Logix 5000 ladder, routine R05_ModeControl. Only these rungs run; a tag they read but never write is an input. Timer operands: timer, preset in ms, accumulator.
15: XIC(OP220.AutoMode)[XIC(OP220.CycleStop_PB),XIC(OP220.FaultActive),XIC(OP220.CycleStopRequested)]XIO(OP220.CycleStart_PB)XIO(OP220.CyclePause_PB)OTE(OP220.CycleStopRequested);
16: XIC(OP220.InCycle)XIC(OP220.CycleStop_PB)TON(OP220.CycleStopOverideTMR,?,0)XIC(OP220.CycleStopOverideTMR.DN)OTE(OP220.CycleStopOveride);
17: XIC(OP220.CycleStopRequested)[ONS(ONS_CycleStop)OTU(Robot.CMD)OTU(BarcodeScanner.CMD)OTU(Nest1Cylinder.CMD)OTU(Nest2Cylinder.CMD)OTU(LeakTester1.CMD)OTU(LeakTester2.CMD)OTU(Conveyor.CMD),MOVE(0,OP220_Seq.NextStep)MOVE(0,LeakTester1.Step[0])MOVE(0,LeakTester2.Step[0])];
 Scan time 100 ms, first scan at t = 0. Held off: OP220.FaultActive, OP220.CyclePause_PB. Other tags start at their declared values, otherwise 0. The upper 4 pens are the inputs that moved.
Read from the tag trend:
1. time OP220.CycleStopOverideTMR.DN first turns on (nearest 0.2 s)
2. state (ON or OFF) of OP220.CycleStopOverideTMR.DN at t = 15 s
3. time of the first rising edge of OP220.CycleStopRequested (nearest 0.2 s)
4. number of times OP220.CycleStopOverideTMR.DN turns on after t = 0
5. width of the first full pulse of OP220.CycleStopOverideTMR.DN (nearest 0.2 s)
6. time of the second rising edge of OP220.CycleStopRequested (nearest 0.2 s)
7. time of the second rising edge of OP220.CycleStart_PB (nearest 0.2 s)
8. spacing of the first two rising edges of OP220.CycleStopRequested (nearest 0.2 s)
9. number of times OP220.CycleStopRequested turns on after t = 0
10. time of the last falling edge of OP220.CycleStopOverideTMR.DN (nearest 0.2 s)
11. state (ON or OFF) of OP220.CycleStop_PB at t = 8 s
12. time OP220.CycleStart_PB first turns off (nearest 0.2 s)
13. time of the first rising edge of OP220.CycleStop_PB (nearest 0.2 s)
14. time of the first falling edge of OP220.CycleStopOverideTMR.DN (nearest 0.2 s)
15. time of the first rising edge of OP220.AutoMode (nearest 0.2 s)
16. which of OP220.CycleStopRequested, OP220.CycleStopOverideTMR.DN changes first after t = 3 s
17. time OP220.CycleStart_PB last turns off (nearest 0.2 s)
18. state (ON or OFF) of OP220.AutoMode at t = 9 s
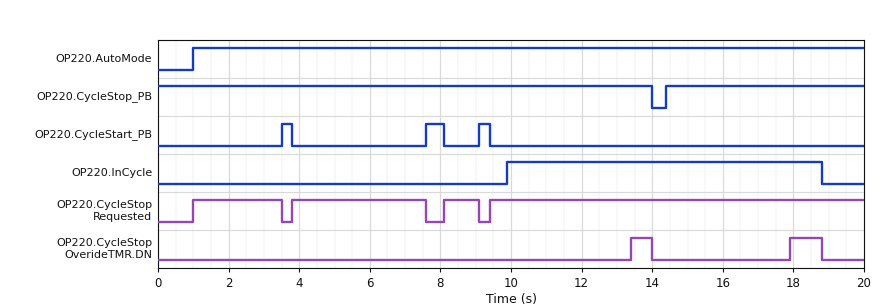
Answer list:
13.4 s
OFF
1.0 s
2
0.6 s
3.8 s
7.6 s
2.8 s
4
18.8 s
ON
3.8 s
14.4 s
14.0 s
1.0 s
OP220.CycleStopRequested
9.4 s
ON
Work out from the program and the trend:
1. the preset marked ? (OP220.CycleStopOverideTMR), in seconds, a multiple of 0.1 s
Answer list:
3.5 s
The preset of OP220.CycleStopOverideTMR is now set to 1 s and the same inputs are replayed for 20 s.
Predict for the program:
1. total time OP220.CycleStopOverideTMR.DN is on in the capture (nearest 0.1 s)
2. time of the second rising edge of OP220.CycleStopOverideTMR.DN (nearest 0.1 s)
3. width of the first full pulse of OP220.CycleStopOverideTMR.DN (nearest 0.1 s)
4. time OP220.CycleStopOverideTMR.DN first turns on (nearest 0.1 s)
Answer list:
6.5 s
15.4 s
3.1 s
10.9 s
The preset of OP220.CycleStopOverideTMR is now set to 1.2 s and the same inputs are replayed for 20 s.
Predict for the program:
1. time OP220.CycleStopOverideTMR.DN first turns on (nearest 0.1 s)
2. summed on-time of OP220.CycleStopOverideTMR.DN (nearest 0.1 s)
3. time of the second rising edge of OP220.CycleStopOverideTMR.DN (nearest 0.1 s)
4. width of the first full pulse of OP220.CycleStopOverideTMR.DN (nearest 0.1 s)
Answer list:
11.1 s
6.1 s
15.6 s
2.9 s
